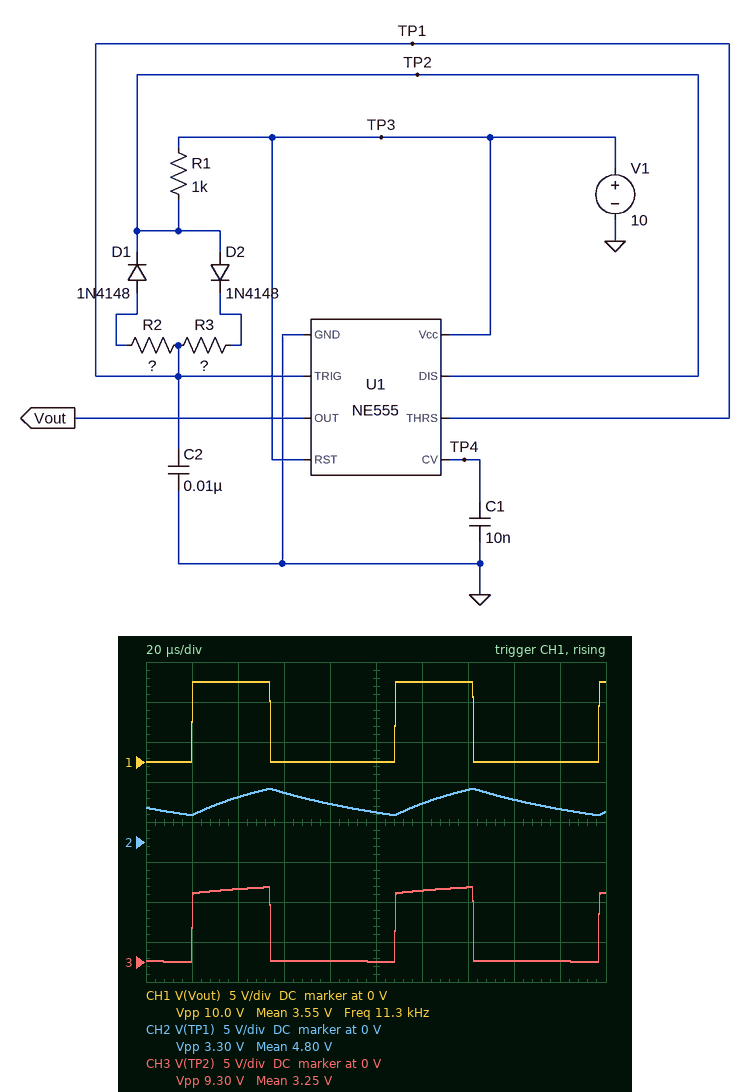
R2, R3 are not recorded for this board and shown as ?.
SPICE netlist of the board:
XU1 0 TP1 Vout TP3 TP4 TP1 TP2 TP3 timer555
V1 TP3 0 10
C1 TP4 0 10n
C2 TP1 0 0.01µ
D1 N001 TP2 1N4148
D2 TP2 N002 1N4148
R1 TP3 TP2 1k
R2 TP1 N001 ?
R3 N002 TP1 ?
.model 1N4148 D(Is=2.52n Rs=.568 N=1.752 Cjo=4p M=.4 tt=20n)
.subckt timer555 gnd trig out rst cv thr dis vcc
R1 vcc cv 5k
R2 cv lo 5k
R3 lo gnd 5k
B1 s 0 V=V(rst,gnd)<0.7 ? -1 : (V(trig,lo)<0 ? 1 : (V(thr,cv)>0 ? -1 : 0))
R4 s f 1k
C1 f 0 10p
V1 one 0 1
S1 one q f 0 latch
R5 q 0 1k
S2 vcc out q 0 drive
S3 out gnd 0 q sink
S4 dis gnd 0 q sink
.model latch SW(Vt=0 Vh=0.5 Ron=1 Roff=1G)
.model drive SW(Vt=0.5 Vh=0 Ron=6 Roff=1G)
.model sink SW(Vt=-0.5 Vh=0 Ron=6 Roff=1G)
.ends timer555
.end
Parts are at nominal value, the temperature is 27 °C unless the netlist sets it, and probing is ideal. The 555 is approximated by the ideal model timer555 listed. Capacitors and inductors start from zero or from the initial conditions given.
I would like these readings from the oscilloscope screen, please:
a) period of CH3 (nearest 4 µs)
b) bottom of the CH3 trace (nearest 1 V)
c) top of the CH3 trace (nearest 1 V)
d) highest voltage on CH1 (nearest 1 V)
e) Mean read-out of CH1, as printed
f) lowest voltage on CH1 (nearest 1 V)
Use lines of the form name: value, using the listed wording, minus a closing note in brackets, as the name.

period of CH3: 88 µs
bottom of the CH3 trace: 0 V
top of the CH3 trace: 9 V
highest voltage on CH1: 10 V
Mean read-out of CH1, as printed: 3.55 V
lowest voltage on CH1: 0 V
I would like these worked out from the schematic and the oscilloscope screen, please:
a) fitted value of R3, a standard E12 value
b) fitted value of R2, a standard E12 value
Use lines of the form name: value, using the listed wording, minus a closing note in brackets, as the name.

fitted value of R3, a standard E12 value: 3.3 kΩ
fitted value of R2, a standard E12 value: 6.8 kΩ
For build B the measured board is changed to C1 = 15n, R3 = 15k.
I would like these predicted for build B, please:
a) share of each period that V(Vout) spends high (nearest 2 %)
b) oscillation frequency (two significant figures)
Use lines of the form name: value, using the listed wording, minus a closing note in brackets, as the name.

share of each period that V(Vout) spends high: 70 %
oscillation frequency: 5.6 kHz
